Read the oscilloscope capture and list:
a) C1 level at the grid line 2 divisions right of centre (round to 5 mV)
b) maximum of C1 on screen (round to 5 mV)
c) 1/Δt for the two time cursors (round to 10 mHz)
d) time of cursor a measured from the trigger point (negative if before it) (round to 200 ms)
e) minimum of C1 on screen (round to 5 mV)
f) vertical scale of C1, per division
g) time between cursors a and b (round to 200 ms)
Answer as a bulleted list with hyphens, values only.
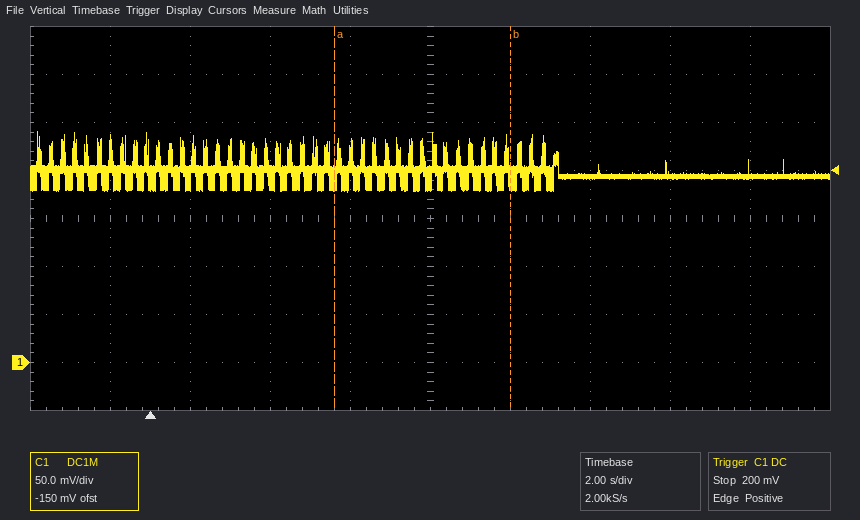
- 195 mV
- 240 mV
- 230 mHz
- +4.6 s
- 180 mV
- 50 mV
- 4.4 s
